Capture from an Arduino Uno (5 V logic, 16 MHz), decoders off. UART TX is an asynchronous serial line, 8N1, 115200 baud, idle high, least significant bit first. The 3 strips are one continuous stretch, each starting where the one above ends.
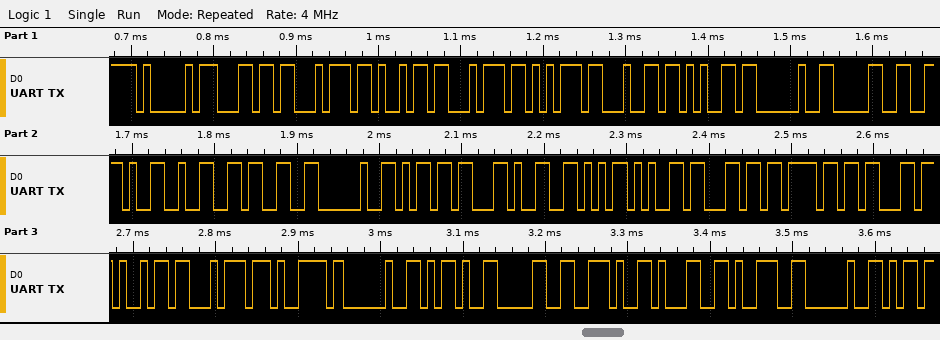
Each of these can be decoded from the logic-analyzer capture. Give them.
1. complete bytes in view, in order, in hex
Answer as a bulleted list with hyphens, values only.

- 41 6C 74 69 74 75 64 65 20 30 2E 32 33 20 6D 2C 56 65 6C 6F 63 69 74 79 20 2D 30 2E 31 39 20
